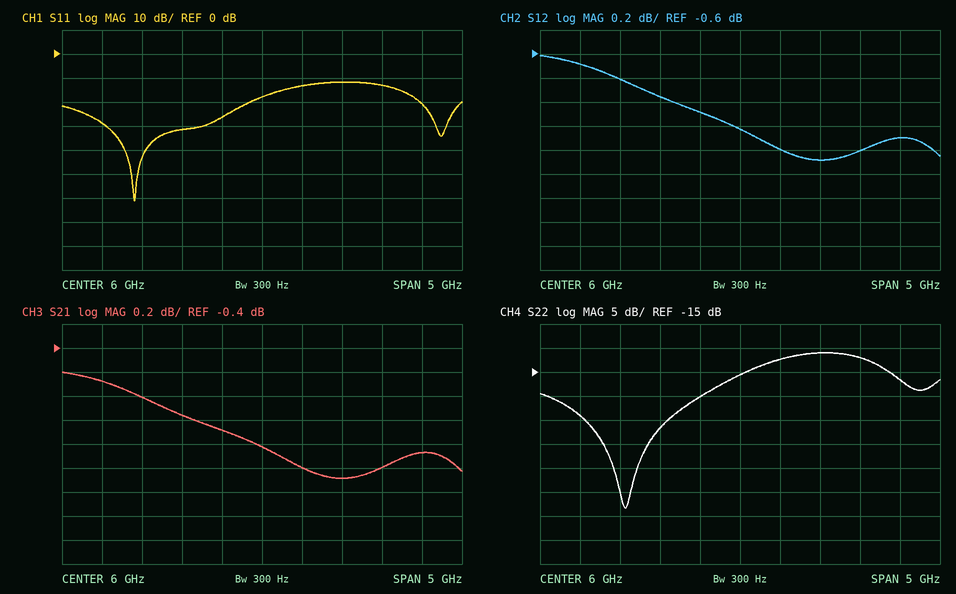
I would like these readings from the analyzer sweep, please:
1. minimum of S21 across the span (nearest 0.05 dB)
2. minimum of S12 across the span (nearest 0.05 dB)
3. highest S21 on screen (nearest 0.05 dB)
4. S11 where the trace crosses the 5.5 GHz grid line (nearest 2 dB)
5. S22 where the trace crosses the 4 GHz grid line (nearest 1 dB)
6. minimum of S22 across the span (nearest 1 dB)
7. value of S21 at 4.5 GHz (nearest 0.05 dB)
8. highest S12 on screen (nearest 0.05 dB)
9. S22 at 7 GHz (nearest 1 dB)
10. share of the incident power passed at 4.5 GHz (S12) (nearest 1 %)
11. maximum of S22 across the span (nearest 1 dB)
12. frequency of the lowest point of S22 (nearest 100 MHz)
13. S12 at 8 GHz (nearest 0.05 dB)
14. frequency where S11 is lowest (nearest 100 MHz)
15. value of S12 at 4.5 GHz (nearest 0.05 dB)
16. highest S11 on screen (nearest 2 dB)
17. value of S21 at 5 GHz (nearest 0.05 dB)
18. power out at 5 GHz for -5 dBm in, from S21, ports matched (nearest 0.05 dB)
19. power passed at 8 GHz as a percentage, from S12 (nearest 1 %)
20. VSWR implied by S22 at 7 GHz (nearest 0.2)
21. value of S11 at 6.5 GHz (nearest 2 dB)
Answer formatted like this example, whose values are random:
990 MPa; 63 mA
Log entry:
-1.50 dB; -1.50 dB; -0.60 dB; -26 dB; -24 dB; -43 dB; -0.80 dB; -0.60 dB; -11 dB; 83 %; -11 dB; 4.6 GHz; -1.30 dB; 4.4 GHz; -0.80 dB; -12 dB; -0.95 dB; -5.95 dBm; 74 %; 1.8; -14 dB
